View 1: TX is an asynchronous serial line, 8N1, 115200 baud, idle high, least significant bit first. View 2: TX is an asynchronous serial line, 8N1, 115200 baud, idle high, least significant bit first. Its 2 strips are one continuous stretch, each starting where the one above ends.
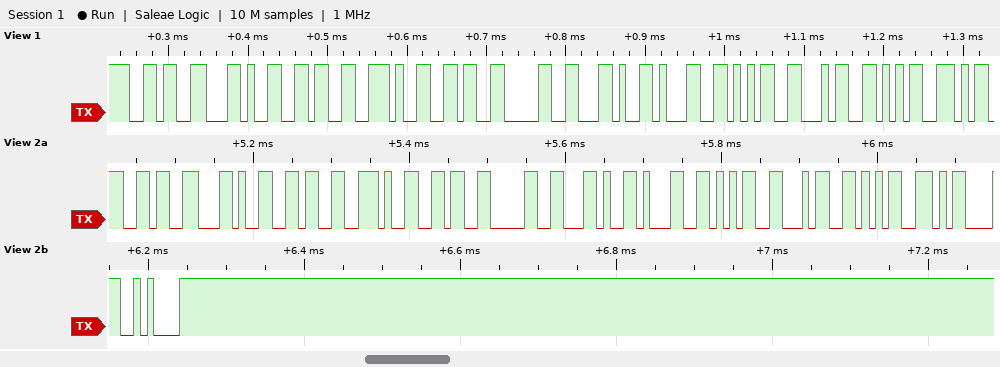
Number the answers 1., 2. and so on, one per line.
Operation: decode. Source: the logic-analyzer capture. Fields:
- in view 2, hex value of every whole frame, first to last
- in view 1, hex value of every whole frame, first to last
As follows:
1. 36 2C 36 2E 36 30 2C 31 35 34 35 0D 0A
2. 0x36 0x2C 0x36 0x2E 0x36 0x30 0x2C 0x31 0x35 0x34 0x35
